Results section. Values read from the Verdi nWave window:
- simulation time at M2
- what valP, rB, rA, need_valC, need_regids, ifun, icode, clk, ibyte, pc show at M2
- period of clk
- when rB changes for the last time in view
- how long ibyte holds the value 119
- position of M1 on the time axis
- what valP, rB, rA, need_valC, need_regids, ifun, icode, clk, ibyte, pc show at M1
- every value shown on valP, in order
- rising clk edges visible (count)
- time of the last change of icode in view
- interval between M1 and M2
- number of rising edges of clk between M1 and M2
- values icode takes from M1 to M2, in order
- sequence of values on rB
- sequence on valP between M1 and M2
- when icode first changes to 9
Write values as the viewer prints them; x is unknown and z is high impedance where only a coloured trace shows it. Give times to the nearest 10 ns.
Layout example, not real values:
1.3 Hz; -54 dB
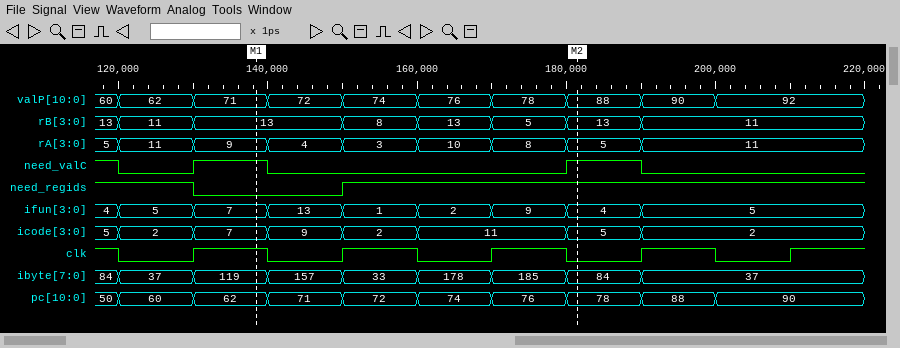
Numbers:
180 ns; valP=88, rB=13, rA=5, need_valC=1, need_regids=1, ifun=4, icode=5, clk=0, ibyte=84, pc=78; 20 ns; 190 ns; 10 ns; 140 ns; valP=71, rB=13, rA=9, need_valC=1, need_regids=0, ifun=7, icode=7, clk=1, ibyte=119, pc=62; 60, 62, 71, 72, 74, 76, 78, 88, 90, 92; 5; 190 ns; 40 ns; 2; 7, 9, 2, 11, 5; 13, 11, 13, 8, 13, 5, 13, 11; 71, 72, 74, 76, 78, 88; 140 ns
